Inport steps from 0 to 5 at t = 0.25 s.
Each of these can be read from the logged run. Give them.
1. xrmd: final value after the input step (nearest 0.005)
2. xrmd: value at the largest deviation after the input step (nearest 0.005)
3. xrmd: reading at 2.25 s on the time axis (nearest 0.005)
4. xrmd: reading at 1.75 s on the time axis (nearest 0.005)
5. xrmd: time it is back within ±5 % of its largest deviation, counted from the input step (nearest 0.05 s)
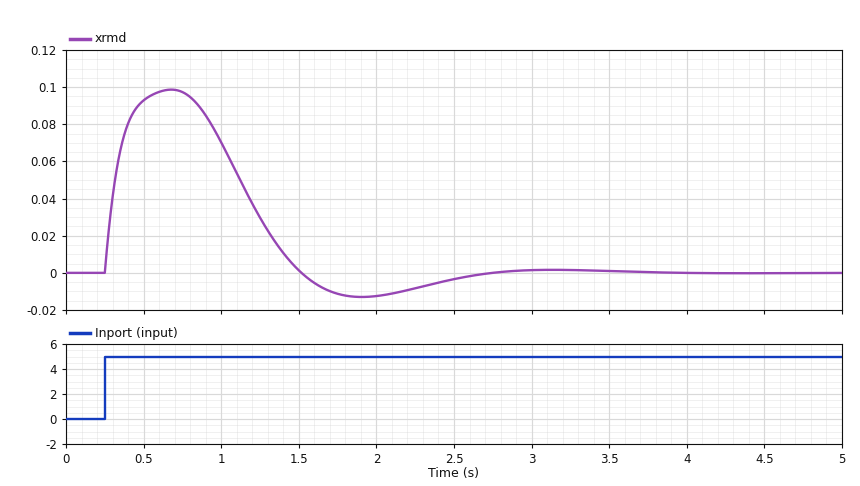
0.000
0.100
-0.010
-0.010
2.15 s
